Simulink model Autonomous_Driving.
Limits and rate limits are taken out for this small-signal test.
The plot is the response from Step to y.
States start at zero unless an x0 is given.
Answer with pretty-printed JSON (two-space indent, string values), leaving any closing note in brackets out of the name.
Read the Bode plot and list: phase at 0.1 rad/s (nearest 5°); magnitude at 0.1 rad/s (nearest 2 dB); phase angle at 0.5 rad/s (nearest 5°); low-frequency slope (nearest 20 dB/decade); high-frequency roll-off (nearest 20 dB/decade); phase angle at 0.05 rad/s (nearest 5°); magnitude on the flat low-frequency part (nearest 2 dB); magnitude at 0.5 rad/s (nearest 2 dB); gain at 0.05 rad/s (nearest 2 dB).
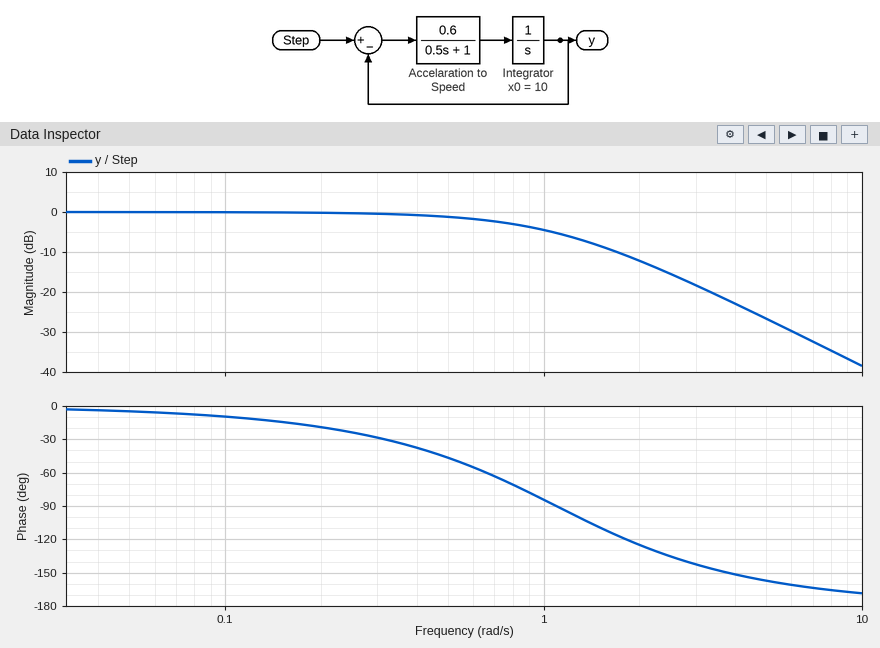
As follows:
{
  "phase at 0.1 rad/s": "-10°",
  "magnitude at 0.1 rad/s": "0 dB",
  "phase angle at 0.5 rad/s": "-45°",
  "low-frequency slope": "0 dB/decade",
  "high-frequency roll-off": "-40 dB/decade",
  "phase angle at 0.05 rad/s": "-5°",
  "magnitude on the flat low-frequency part": "0 dB",
  "magnitude at 0.5 rad/s": "-2 dB",
  "gain at 0.05 rad/s": "0 dB"
}
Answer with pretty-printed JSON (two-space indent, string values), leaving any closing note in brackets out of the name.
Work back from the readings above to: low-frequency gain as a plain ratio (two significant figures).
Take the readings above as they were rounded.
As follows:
{
  "low-frequency gain as a plain ratio": "1.0"
}
